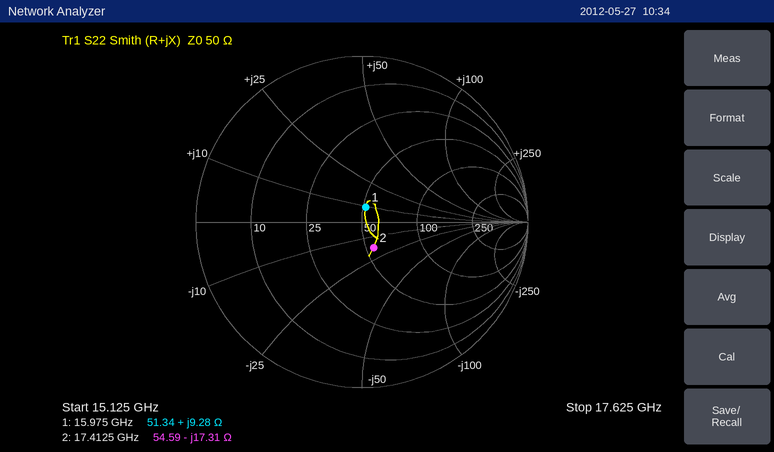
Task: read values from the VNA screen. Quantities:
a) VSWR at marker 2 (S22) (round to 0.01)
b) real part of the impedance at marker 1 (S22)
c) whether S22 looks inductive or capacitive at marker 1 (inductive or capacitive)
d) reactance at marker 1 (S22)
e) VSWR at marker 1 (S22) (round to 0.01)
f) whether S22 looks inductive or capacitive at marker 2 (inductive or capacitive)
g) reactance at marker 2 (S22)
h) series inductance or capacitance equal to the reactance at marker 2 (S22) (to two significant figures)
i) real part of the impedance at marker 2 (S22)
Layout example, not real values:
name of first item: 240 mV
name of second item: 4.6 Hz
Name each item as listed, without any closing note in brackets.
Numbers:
VSWR at marker 2 (S22): 1.41
real part of the impedance at marker 1: 51.34 Ω
whether S22 looks inductive or capacitive at marker 1: inductive
reactance at marker 1: +9.28 Ω
VSWR at marker 1 (S22): 1.20
whether S22 looks inductive or capacitive at marker 2: capacitive
reactance at marker 2: -17.31 Ω
series inductance or capacitance equal to the reactance at marker 2 (S22): 530 fF
real part of the impedance at marker 2: 54.59 Ω
